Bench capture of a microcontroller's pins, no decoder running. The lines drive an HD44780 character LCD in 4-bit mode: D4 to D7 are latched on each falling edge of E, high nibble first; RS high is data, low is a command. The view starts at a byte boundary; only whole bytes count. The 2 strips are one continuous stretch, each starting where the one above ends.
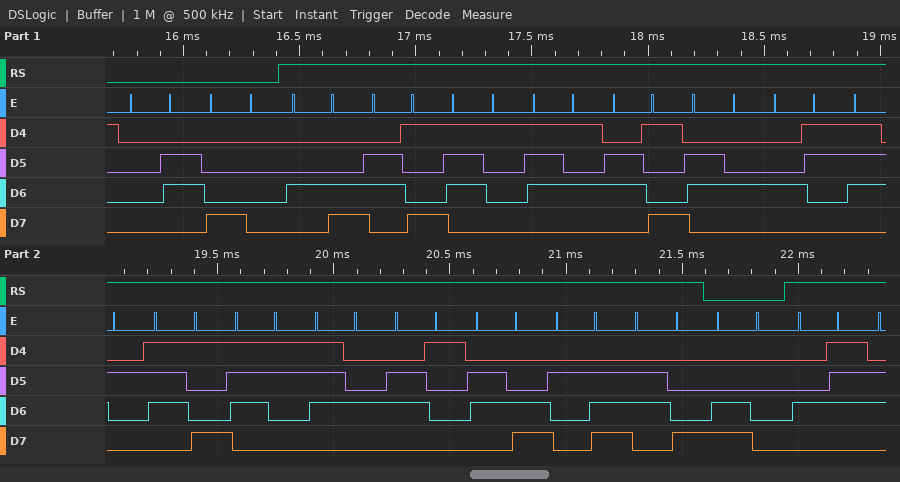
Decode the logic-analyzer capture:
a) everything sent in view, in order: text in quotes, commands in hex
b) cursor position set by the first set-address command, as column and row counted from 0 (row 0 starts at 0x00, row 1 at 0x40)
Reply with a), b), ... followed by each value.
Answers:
a) 0x06 0x80 "LiquidCrystal.h" 0xC0 "G"
b) column 0, row 0
